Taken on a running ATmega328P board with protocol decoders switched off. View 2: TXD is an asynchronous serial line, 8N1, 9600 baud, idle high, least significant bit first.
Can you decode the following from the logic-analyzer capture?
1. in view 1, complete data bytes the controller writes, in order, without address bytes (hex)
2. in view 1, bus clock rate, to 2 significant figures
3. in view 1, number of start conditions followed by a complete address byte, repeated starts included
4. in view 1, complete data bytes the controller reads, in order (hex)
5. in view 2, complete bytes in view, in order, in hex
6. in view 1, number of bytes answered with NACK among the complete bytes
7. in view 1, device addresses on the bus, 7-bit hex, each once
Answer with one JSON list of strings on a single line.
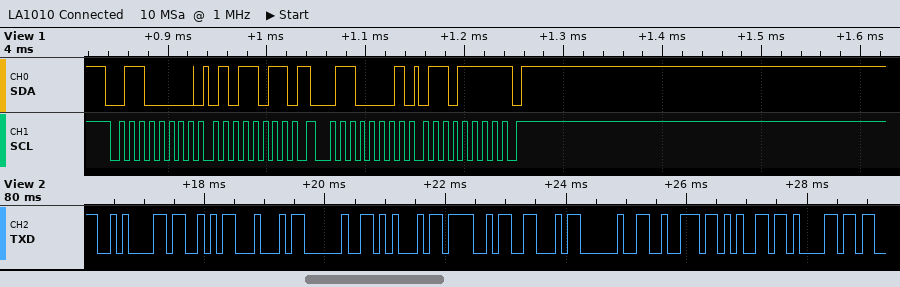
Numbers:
["5B", "100 kHz", "2", "6F", "0A 53 44 20 45 4F 46 20 72 65 61", "1", "0x30"]
